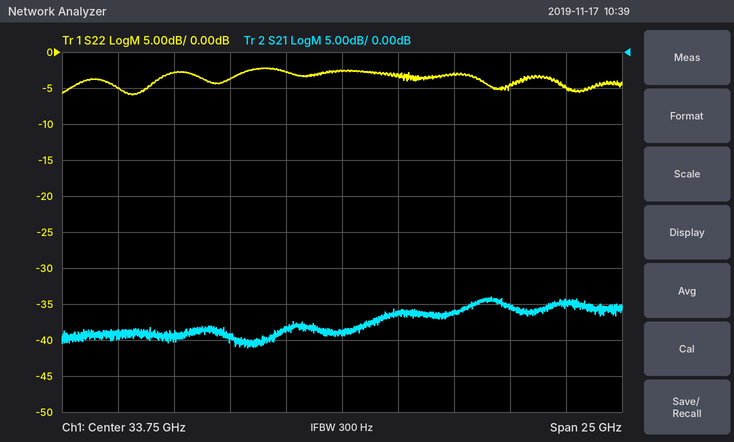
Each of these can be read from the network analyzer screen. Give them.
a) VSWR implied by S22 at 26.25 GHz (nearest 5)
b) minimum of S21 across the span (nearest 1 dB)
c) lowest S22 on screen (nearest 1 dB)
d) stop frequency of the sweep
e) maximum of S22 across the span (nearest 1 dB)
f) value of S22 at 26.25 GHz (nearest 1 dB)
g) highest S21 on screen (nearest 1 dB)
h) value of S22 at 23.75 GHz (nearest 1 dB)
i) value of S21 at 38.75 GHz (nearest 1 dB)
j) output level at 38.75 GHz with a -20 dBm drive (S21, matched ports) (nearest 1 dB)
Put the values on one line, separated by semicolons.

5; -41 dB; -6 dB; 46.25 GHz; -2 dB; -3 dB; -34 dB; -5 dB; -36 dB; -56 dBm
